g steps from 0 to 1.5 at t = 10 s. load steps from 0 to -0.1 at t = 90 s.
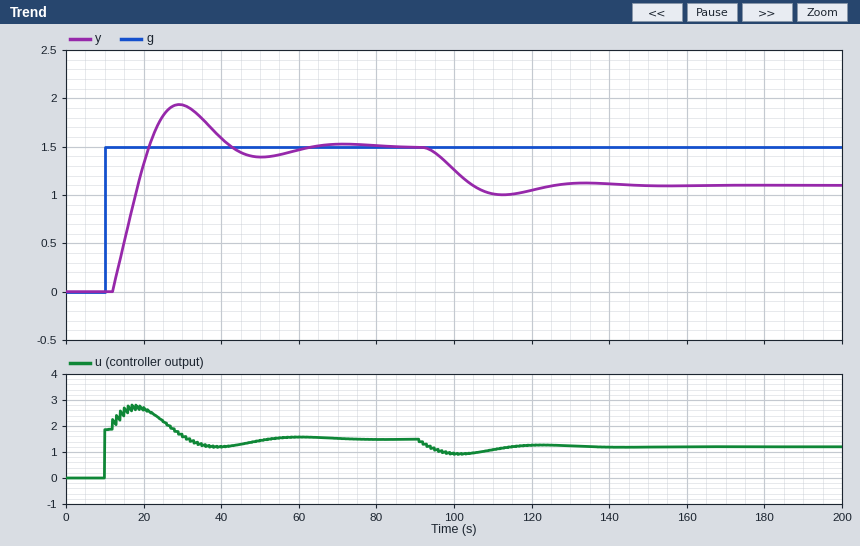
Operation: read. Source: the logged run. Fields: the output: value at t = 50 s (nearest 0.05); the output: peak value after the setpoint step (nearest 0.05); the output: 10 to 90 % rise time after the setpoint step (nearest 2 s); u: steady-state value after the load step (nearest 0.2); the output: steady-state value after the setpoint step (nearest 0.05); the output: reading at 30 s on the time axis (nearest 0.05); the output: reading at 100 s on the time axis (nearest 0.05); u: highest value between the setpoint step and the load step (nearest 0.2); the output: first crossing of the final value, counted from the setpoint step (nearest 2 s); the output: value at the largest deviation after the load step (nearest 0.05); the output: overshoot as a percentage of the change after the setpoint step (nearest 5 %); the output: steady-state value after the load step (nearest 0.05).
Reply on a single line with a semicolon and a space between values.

1.40; 1.95; 8 s; 1.2; 1.50; 1.95; 1.25; 2.8; 12 s; 1.00; 30 %; 1.10
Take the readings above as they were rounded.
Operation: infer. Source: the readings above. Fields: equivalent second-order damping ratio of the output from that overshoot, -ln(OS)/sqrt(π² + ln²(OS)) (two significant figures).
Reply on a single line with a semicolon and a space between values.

0.36
